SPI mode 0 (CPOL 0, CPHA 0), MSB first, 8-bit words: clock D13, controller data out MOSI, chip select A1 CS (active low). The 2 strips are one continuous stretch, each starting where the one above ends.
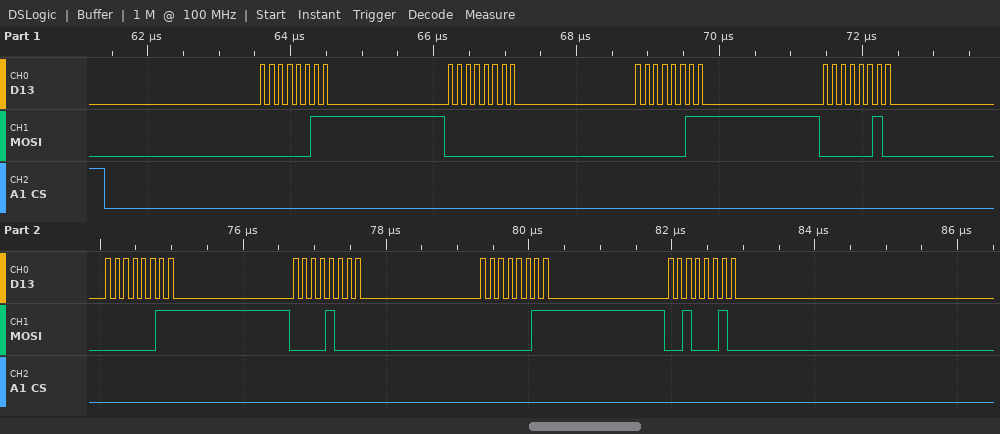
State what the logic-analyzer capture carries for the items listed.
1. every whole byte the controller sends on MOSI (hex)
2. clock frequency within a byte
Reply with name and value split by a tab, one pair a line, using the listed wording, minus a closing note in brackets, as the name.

every whole byte the controller sends on MOSI	03 00 03 02 03 08 03 22
clock frequency within a byte	8 MHz
